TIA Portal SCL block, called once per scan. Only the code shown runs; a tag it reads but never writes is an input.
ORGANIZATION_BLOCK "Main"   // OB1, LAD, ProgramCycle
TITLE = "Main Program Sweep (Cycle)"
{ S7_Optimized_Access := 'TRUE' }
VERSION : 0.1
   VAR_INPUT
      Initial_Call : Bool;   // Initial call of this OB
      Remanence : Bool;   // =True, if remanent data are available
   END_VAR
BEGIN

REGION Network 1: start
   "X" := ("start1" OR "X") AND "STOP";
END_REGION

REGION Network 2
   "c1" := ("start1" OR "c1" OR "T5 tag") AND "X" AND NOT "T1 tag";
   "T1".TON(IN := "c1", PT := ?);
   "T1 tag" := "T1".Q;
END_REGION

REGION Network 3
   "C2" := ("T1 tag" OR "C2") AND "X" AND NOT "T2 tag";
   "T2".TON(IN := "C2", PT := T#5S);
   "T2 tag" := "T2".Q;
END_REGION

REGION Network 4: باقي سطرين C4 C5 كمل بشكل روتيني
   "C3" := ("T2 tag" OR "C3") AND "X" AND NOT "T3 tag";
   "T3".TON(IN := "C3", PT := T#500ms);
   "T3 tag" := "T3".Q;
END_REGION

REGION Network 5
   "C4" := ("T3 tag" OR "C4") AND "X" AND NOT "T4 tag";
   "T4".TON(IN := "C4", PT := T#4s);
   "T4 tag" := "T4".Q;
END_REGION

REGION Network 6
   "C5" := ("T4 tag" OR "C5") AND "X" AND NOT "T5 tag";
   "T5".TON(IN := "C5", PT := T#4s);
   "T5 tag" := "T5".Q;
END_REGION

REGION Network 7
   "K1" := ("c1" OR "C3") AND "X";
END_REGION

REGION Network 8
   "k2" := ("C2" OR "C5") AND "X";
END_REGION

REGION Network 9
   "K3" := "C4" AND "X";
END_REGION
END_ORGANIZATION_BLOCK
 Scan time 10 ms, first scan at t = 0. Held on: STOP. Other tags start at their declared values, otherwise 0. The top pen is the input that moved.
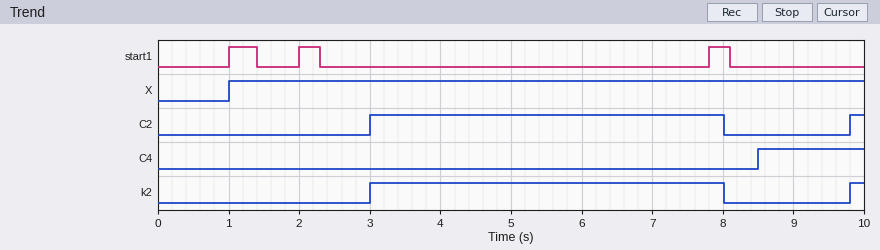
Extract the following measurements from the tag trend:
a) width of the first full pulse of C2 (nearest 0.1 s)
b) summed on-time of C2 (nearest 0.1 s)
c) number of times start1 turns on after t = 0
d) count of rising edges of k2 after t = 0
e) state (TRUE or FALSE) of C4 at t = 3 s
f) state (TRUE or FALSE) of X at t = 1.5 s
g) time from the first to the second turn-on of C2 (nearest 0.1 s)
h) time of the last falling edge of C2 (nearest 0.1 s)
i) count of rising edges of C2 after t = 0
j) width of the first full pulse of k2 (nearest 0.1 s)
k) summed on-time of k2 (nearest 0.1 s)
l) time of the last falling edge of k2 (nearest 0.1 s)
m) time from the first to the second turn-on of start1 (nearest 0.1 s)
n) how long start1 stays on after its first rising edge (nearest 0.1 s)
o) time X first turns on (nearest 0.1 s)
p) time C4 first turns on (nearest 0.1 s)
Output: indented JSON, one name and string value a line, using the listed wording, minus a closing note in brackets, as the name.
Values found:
{
  "width of the first full pulse of C2": "5.0 s",
  "summed on-time of C2": "5.2 s",
  "number of times start1 turns on after t = 0": "3",
  "count of rising edges of k2 after t = 0": "2",
  "state (TRUE or FALSE) of C4 at t = 3 s": "FALSE",
  "state (TRUE or FALSE) of X at t = 1.5 s": "TRUE",
  "time from the first to the second turn-on of C2": "6.8 s",
  "time of the last falling edge of C2": "8.0 s",
  "count of rising edges of C2 after t = 0": "2",
  "width of the first full pulse of k2": "5.0 s",
  "summed on-time of k2": "5.2 s",
  "time of the last falling edge of k2": "8.0 s",
  "time from the first to the second turn-on of start1": "1.0 s",
  "how long start1 stays on after its first rising edge": "0.4 s",
  "time X first turns on": "1.0 s",
  "time C4 first turns on": "8.5 s"
}
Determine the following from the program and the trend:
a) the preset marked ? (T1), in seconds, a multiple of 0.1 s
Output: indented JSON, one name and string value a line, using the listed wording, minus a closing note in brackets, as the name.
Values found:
{
  "the preset marked ? (T1), in seconds, a multiple of 0.1 s": "2.0 s"
}
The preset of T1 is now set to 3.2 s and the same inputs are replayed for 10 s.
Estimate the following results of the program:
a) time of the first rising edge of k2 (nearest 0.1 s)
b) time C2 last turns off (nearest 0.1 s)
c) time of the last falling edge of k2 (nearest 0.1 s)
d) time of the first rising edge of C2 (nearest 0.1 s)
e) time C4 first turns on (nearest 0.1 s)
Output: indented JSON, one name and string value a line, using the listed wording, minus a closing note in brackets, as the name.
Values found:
{
  "time of the first rising edge of k2": "4.2 s",
  "time C2 last turns off": "9.2 s",
  "time of the last falling edge of k2": "9.2 s",
  "time of the first rising edge of C2": "4.2 s",
  "time C4 first turns on": "9.7 s"
}
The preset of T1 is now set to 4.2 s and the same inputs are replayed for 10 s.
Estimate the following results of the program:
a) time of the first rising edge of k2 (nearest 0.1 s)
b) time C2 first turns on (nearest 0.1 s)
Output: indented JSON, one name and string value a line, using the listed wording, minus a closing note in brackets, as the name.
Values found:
{
  "time of the first rising edge of k2": "5.2 s",
  "time C2 first turns on": "5.2 s"
}
